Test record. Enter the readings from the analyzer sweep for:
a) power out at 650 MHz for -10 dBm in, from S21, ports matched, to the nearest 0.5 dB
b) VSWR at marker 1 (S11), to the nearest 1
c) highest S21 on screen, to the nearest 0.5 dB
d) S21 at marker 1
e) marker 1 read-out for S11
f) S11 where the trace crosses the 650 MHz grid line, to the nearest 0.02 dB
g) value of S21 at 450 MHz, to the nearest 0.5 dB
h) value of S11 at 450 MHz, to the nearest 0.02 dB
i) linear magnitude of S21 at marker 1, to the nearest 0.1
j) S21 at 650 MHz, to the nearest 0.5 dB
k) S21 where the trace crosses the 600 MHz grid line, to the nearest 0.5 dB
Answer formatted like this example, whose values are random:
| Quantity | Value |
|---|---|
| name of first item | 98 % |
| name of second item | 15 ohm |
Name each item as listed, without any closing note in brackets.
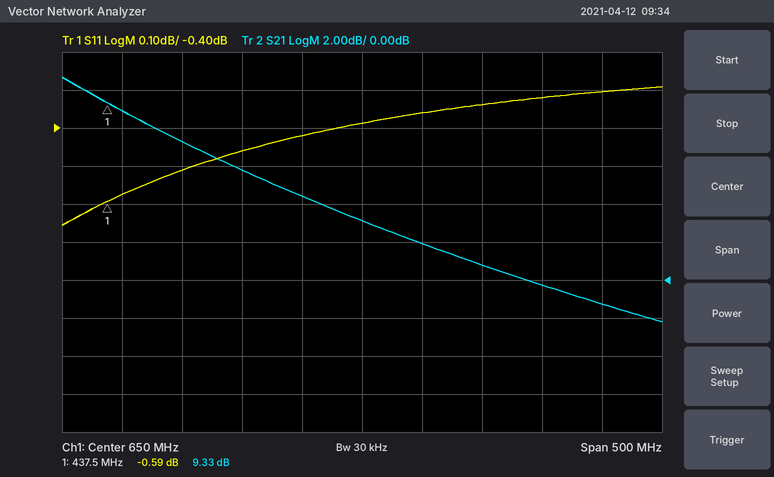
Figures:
| Quantity | Value |
|---|---|
| power out at 650 MHz for -10 dBm in, from S21, ports matched, to the nearest 0.5 dB | -7.0 dBm |
| VSWR at marker 1 (S11), to the nearest 1 | 29 |
| highest S21 on screen, to the nearest 0.5 dB | 10.5 dB |
| S21 at marker 1 | 9.33 dB |
| marker 1 read-out for S11 | -0.59 dB |
| S11 where the trace crosses the 650 MHz grid line, to the nearest 0.02 dB | -0.38 dB |
| value of S21 at 450 MHz, to the nearest 0.5 dB | 9.0 dB |
| value of S11 at 450 MHz, to the nearest 0.02 dB | -0.58 dB |
| linear magnitude of S21 at marker 1, to the nearest 0.1 | 2.9 |
| S21 at 650 MHz, to the nearest 0.5 dB | 3.0 dB |
| S21 where the trace crosses the 600 MHz grid line, to the nearest 0.5 dB | 4.5 dB |
